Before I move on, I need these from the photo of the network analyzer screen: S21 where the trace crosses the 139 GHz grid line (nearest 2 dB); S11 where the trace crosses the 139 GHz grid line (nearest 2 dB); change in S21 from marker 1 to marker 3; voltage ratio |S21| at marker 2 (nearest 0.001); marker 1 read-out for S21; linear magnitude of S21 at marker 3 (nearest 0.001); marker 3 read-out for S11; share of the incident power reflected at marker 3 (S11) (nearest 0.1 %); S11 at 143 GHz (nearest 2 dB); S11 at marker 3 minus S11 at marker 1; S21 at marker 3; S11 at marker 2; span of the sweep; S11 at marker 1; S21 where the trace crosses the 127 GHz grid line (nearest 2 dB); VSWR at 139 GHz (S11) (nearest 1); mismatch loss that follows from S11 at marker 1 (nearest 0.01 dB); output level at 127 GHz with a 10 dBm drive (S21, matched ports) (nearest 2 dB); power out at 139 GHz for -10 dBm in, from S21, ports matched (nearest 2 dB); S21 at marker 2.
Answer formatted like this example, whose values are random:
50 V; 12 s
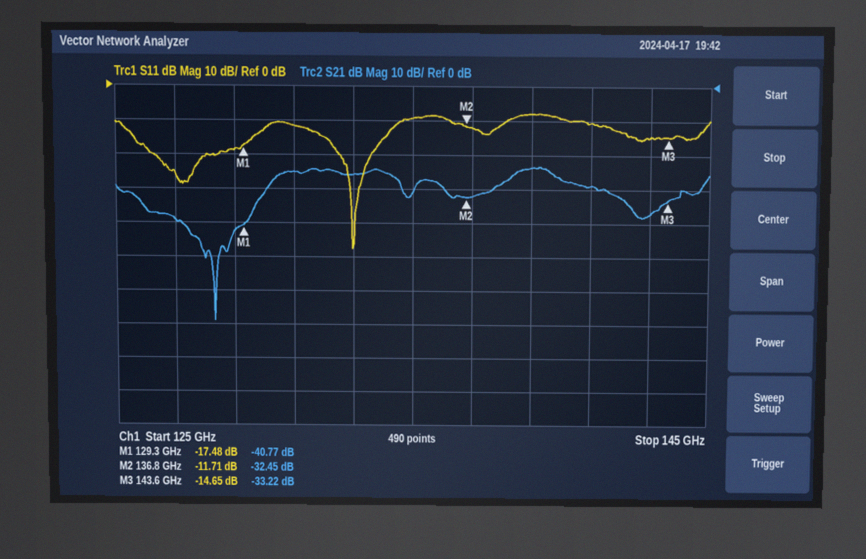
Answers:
-24 dB; -8 dB; 7.55 dB; 0.024; -40.77 dB; 0.022; -14.65 dB; 3.4 %; -14 dB; 2.83 dB; -33.22 dB; -11.71 dB; 20 GHz; -17.48 dB; -40 dB; 2; 0.08 dB; -30 dBm; -34 dBm; -32.45 dB
